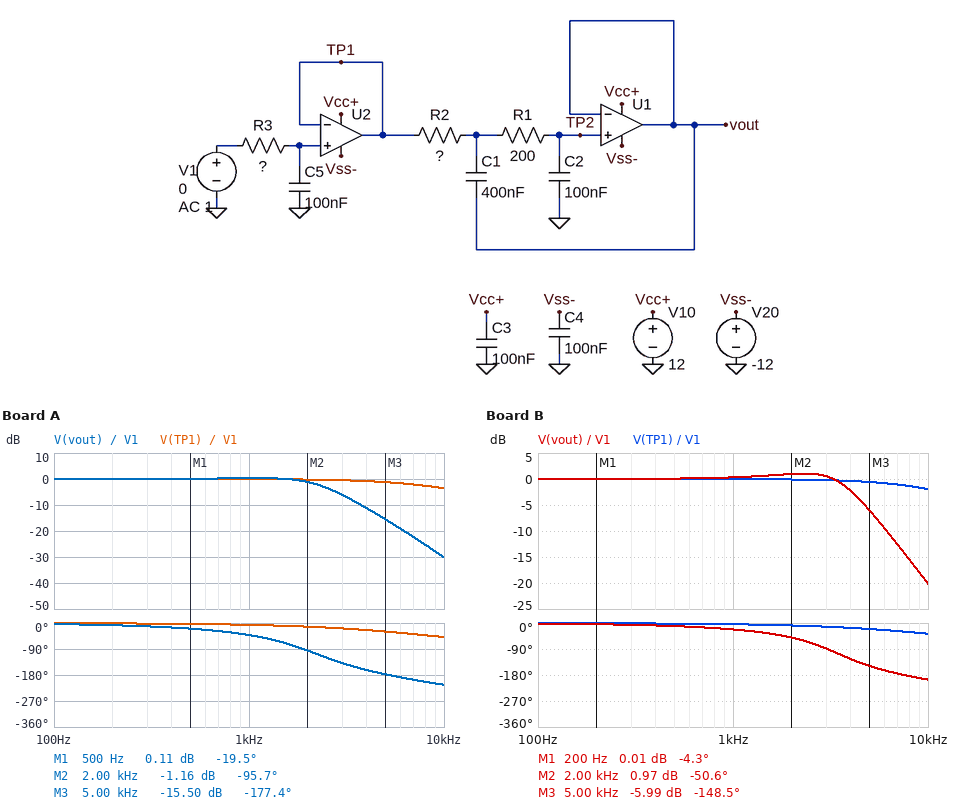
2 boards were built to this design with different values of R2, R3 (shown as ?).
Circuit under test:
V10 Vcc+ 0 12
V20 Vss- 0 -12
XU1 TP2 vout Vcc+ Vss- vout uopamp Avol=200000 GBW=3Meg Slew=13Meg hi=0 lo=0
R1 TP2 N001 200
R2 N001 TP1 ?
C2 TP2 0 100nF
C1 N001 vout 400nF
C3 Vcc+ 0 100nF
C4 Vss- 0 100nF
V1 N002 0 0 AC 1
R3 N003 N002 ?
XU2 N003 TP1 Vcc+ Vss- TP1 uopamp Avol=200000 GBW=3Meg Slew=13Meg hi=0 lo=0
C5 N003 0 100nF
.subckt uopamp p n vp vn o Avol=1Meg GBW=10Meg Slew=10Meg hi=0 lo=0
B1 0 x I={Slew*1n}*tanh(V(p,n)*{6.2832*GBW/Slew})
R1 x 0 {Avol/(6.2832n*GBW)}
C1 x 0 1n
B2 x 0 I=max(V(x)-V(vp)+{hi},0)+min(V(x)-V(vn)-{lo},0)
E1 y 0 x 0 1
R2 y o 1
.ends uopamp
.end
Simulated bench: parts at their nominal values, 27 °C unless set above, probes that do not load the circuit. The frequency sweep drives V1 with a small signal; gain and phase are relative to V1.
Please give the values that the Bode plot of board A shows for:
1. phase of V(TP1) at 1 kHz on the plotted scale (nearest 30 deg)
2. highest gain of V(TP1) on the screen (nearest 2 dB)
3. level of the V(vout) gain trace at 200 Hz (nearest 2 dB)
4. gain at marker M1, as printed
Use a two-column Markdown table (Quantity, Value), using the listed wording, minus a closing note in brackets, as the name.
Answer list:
| Quantity | Value |
|---|---|
| phase of V(TP1) at 1 kHz on the plotted scale | 0 deg |
| highest gain of V(TP1) on the screen | 0 dB |
| level of the V(vout) gain trace at 200 Hz | 0 dB |
| gain at marker M1, as printed | 0.11 dB |
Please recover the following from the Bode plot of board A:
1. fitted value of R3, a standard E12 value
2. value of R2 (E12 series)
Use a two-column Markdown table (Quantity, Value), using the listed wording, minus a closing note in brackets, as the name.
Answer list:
| Quantity | Value |
|---|---|
| fitted value of R3, a standard E12 value | 180 Ω |
| value of R2 | 680 Ω |
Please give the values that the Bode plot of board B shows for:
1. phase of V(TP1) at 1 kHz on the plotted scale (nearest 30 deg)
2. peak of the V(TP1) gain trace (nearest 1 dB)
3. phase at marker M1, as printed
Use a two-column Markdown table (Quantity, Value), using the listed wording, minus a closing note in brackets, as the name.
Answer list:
| Quantity | Value |
|---|---|
| phase of V(TP1) at 1 kHz on the plotted scale | 0 deg |
| peak of the V(TP1) gain trace | 0 dB |
| phase at marker M1, as printed | -4.3 deg |
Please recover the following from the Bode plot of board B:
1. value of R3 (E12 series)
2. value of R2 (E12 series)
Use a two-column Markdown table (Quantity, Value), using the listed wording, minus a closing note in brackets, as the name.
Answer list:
| Quantity | Value |
|---|---|
| value of R3 | 120 Ω |
| value of R2 | 270 Ω |
